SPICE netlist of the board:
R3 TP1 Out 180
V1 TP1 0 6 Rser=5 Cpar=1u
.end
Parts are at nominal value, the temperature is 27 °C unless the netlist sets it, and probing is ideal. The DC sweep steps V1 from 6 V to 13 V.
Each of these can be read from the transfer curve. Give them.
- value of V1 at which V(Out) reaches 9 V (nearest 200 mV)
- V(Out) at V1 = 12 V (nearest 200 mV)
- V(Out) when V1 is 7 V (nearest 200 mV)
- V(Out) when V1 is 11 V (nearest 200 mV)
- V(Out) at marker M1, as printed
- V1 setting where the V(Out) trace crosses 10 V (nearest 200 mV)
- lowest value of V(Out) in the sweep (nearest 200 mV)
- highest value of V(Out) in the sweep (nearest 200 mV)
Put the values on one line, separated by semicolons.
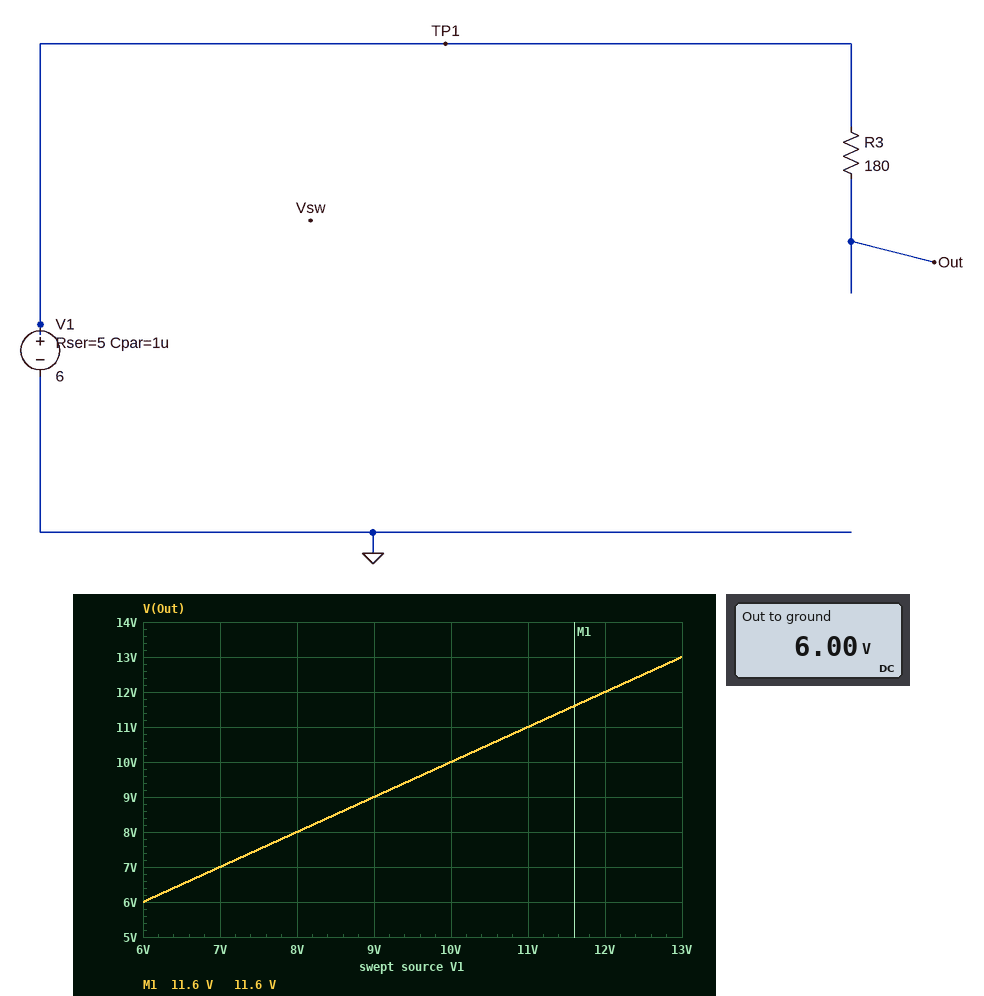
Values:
9.0 V; 12.0 V; 7.0 V; 11.0 V; 11.6 V; 10.0 V; 6.0 V; 13.0 V
